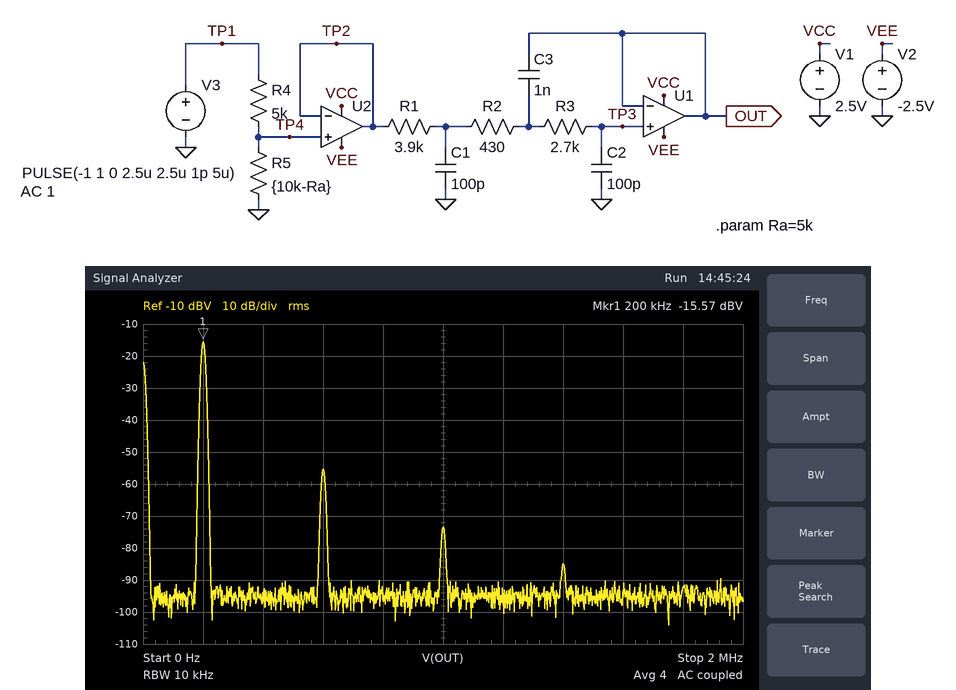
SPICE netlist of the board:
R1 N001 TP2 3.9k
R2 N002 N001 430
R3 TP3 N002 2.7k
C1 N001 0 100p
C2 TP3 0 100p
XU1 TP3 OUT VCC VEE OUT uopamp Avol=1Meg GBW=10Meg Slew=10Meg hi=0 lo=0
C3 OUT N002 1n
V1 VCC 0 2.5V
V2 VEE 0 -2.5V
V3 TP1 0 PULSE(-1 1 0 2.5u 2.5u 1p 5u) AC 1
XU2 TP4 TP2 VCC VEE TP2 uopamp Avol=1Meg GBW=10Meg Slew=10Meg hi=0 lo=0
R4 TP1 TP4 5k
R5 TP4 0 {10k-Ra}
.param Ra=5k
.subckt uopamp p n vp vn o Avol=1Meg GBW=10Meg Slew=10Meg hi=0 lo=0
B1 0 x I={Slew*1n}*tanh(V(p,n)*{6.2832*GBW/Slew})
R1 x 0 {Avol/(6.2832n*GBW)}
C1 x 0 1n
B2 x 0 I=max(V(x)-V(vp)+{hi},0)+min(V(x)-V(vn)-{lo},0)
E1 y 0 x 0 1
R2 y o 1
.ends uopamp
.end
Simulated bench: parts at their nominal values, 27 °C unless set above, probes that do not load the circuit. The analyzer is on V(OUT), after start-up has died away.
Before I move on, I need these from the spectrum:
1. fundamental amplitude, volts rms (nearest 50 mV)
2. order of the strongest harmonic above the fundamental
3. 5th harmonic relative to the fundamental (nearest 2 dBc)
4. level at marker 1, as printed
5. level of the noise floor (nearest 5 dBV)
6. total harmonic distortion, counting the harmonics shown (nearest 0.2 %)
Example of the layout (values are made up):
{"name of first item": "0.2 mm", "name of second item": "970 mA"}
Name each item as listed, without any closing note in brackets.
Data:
{"fundamental amplitude, volts rms": "150 mV", "order of the strongest harmonic above the fundamental": "3", "5th harmonic relative to the fundamental": "-58 dBc", "level at marker 1, as printed": "-15.57 dBV", "level of the noise floor": "-95 dBV", "total harmonic distortion, counting the harmonics shown": "1.0 %"}
